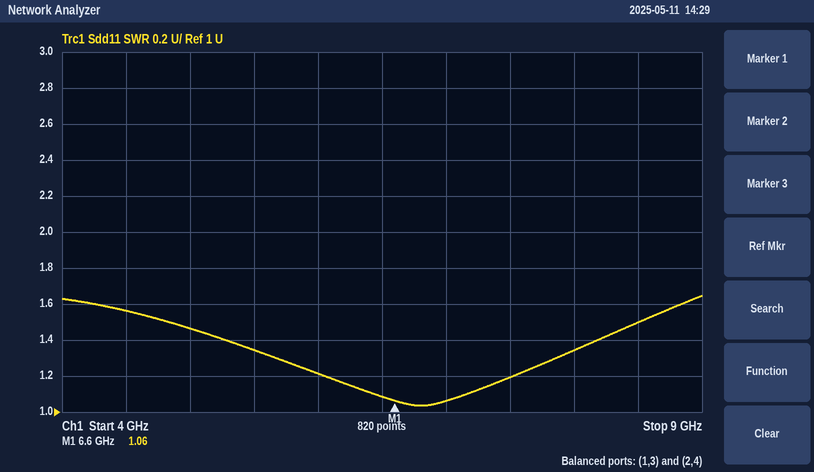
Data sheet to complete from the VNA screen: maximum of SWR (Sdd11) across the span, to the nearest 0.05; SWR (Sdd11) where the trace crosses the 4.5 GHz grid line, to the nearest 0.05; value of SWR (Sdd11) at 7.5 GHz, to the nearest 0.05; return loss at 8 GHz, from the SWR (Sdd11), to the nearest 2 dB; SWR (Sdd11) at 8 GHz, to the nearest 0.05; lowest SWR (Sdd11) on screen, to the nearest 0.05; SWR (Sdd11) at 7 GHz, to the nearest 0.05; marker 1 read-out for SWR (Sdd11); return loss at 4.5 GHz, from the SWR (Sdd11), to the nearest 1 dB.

1.65
1.55
1.20
16 dB
1.35
1.05
1.05
1.06
13 dB
